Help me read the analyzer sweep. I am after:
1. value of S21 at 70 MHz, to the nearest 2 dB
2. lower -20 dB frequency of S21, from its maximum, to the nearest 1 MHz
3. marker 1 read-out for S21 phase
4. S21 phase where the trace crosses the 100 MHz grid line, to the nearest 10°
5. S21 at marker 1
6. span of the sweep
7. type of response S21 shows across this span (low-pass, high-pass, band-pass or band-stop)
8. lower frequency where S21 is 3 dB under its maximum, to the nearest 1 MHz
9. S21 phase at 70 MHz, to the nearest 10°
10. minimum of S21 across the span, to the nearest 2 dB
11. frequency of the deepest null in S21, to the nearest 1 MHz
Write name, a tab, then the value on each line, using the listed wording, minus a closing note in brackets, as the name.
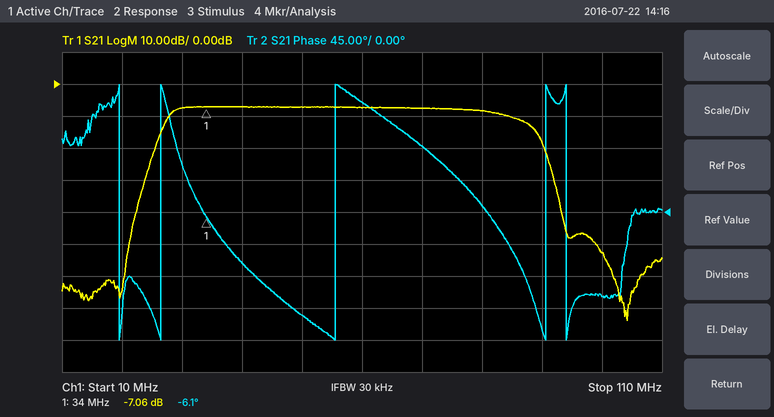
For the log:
value of S21 at 70 MHz, to the nearest 2 dB	-8 dB
lower -20 dB frequency of S21, from its maximum, to the nearest 1 MHz	24 MHz
marker 1 read-out for S21 phase	-6.1°
S21 phase where the trace crosses the 100 MHz grid line, to the nearest 10°	-120°
S21 at marker 1	-7.06 dB
span of the sweep	100 MHz
type of response S21 shows across this span	band-pass
lower frequency where S21 is 3 dB under its maximum, to the nearest 1 MHz	28 MHz
S21 phase at 70 MHz, to the nearest 10°	90°
minimum of S21 across the span, to the nearest 2 dB	-74 dB
frequency of the deepest null in S21, to the nearest 1 MHz	104 MHz
